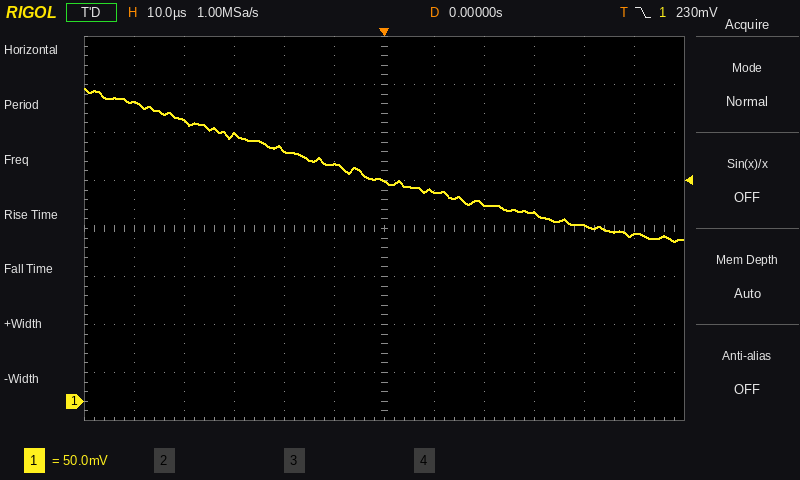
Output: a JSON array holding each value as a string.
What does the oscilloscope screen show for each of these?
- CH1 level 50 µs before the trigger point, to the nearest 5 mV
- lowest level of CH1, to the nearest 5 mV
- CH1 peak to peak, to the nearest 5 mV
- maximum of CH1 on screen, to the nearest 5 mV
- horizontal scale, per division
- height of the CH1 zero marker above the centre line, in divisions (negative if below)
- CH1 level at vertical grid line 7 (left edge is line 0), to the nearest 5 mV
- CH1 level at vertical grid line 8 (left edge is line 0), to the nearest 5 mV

["310 mV", "165 mV", "160 mV", "325 mV", "10 µs", "-3.6 div", "220 mV", "205 mV"]
